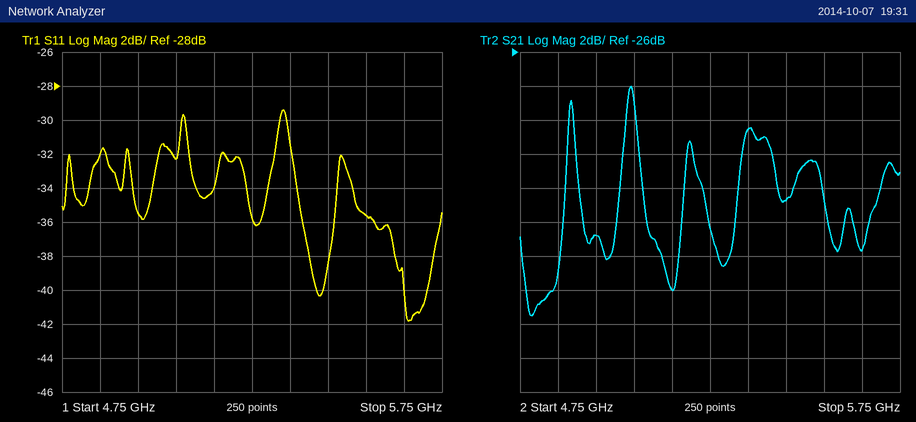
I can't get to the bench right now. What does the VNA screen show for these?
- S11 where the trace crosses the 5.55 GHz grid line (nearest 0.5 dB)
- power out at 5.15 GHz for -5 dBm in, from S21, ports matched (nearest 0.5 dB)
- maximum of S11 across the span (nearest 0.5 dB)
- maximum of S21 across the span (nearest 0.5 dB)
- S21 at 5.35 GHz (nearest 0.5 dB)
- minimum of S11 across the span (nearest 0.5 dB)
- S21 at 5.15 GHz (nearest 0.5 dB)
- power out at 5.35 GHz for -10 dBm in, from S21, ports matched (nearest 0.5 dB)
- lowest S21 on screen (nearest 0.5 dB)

-35.5 dB
-45.0 dBm
-29.5 dB
-28.0 dB
-30.5 dB
-42.0 dB
-40.0 dB
-40.5 dBm
-41.5 dB
